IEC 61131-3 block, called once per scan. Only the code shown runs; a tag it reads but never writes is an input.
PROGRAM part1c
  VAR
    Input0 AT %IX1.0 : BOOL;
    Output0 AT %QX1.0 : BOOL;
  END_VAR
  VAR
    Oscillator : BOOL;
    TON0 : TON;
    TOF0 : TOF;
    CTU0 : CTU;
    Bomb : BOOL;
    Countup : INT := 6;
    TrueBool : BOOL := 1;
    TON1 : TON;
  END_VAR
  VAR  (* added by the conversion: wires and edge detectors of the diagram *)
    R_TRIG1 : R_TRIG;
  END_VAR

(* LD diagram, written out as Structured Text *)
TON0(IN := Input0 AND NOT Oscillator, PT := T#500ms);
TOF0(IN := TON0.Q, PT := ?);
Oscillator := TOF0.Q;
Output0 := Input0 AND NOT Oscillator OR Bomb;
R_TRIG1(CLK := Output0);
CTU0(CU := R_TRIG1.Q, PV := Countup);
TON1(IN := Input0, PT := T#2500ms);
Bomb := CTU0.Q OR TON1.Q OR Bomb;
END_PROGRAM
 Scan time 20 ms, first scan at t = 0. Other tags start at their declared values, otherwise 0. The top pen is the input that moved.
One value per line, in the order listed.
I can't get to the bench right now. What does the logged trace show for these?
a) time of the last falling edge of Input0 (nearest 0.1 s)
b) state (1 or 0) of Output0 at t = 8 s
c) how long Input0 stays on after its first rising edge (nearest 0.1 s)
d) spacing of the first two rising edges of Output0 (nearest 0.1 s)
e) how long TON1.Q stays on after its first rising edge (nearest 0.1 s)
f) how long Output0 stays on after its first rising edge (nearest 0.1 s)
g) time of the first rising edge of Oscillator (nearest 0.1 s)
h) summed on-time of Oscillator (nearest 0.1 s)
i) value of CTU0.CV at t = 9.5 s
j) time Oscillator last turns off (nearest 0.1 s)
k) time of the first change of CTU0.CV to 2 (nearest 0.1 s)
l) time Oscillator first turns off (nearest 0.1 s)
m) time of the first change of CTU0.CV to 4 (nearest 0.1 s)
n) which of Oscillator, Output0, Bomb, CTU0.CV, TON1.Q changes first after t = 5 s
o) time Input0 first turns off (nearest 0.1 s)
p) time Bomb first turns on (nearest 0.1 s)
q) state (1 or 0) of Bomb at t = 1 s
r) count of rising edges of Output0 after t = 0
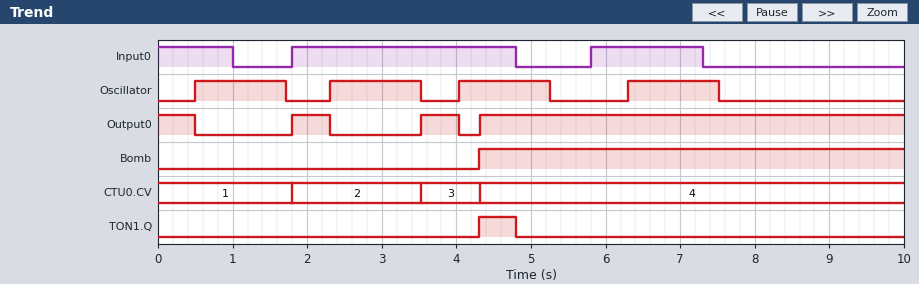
7.3 s
1
3.0 s
1.7 s
0.5 s
0.5 s
0.5 s
4.9 s
4
7.5 s
1.8 s
1.7 s
4.3 s
Oscillator
1.0 s
4.3 s
0
3
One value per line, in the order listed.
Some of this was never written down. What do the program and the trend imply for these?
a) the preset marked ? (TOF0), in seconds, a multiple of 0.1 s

1.2 s
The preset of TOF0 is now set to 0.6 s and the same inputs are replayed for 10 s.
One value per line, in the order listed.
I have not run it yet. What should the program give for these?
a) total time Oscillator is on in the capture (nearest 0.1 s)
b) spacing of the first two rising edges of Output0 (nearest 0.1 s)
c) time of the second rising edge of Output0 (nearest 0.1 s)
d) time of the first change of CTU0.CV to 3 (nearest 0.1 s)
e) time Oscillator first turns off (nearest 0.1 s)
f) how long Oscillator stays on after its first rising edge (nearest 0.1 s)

3.1 s
1.1 s
2.9 s
2.9 s
1.1 s
0.6 s
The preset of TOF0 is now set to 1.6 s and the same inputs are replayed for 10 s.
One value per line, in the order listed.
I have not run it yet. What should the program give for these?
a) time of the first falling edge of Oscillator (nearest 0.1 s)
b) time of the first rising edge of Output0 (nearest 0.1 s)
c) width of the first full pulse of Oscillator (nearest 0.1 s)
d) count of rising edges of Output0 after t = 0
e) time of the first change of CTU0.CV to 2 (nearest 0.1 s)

2.1 s
2.1 s
1.6 s
2
2.1 s
